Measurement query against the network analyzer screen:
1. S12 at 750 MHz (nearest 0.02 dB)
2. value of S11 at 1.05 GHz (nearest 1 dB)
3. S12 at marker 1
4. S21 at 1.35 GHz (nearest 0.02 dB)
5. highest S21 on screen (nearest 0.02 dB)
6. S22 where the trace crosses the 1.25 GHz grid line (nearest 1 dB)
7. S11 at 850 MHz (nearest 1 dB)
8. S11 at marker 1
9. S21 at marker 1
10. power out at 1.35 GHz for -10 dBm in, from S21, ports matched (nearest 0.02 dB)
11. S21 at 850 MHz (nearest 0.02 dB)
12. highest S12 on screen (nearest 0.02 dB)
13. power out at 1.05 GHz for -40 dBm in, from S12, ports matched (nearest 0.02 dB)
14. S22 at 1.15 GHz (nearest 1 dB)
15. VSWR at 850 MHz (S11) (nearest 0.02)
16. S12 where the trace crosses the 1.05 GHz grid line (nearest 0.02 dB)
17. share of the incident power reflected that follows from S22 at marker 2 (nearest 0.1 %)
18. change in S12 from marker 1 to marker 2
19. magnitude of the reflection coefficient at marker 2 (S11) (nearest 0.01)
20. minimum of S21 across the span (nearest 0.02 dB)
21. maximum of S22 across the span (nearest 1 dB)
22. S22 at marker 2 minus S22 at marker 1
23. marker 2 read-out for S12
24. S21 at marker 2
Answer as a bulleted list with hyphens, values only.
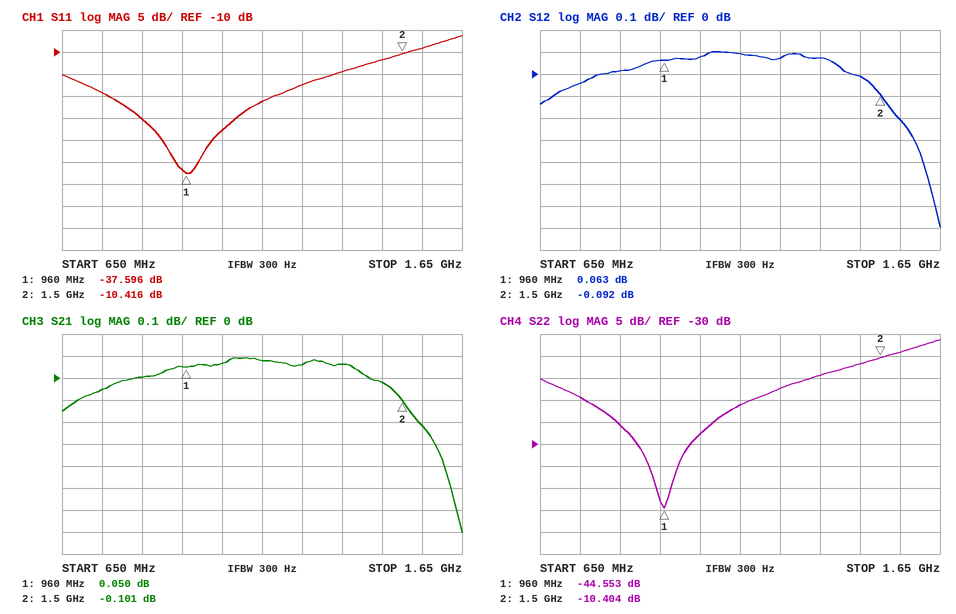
- -0.04 dB
- -28 dB
- 0.063 dB
- 0.06 dB
- 0.10 dB
- -17 dB
- -25 dB
- -37.596 dB
- 0.050 dB
- -9.94 dBm
- 0.00 dB
- 0.10 dB
- -39.92 dBm
- -21 dB
- 1.12
- 0.08 dB
- 9.1 %
- -0.155 dB
- 0.30
- -0.70 dB
- -6 dB
- 34.149 dB
- -0.092 dB
- -0.101 dB
